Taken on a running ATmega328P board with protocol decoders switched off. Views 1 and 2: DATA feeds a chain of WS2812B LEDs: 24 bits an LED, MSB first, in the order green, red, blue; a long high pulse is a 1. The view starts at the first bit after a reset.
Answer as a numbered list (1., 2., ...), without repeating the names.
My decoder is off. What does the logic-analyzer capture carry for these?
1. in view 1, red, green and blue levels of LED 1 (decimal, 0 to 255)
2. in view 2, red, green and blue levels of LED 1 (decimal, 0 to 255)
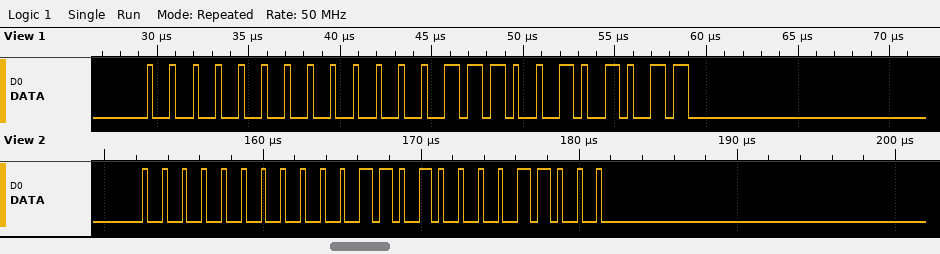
1. 7, 0, 43
2. 26, 0, 24
